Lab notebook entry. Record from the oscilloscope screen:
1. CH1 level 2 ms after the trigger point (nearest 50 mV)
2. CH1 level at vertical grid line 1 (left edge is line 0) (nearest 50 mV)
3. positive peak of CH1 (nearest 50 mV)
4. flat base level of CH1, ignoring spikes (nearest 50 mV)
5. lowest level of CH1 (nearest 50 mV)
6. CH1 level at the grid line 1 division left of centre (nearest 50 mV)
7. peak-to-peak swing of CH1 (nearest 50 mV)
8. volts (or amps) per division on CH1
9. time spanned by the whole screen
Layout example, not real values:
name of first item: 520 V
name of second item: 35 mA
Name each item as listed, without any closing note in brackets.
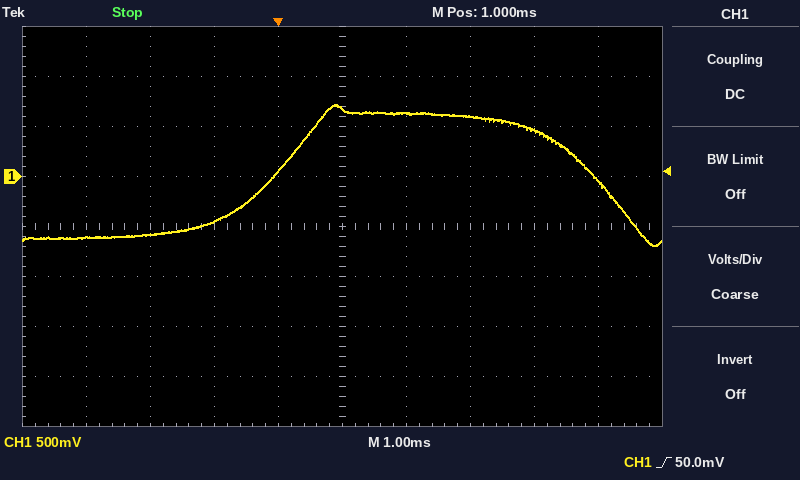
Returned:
CH1 level 2 ms after the trigger point: 650 mV
CH1 level at vertical grid line 1 (left edge is line 0): -600 mV
positive peak of CH1: 700 mV
flat base level of CH1, ignoring spikes: -600 mV
lowest level of CH1: -700 mV
CH1 level at the grid line 1 division left of centre: 50 mV
peak-to-peak swing of CH1: 1.40 V
volts (or amps) per division on CH1: 500 mV
time spanned by the whole screen: 10 ms
